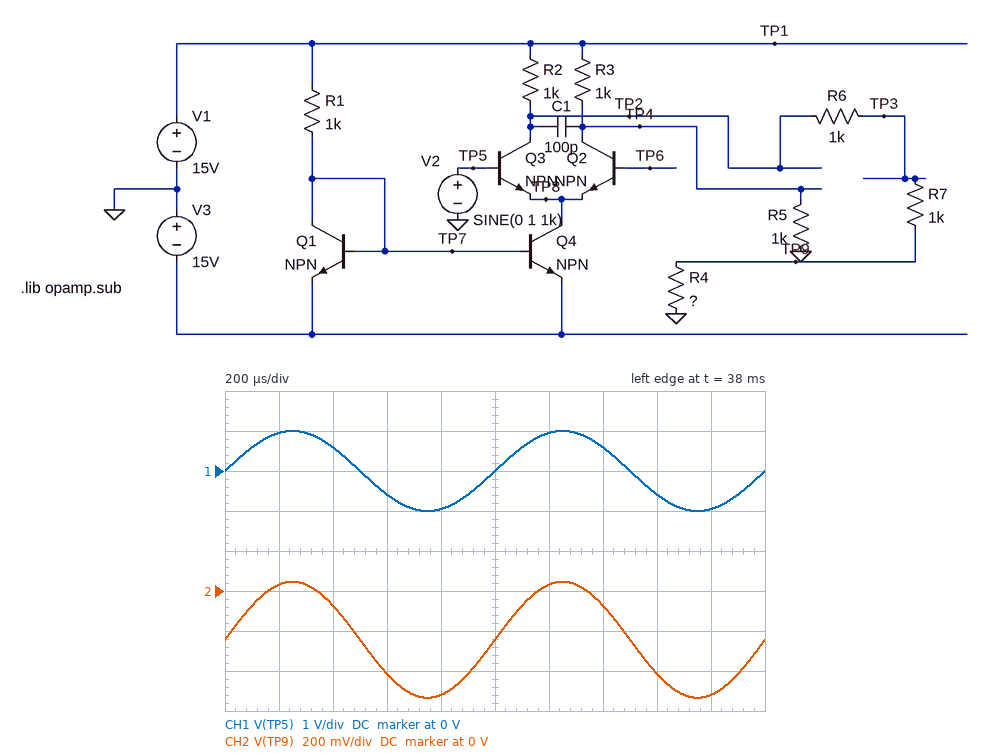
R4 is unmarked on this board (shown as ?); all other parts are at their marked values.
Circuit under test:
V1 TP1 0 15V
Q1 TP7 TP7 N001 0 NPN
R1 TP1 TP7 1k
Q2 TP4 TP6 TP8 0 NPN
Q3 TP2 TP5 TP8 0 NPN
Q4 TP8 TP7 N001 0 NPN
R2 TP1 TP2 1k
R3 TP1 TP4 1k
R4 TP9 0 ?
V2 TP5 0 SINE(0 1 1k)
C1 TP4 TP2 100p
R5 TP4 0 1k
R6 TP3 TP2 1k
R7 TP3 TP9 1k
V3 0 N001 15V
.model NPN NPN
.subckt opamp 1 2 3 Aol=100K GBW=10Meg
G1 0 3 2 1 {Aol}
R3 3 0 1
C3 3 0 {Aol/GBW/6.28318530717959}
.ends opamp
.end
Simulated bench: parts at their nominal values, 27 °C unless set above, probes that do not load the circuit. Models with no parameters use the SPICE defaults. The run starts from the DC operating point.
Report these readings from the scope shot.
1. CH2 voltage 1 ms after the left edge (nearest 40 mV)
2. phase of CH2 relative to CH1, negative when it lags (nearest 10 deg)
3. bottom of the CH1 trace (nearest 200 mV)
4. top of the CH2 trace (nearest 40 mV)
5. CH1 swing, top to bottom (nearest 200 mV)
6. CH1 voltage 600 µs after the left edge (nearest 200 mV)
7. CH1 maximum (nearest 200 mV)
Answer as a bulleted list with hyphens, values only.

- -240 mV
- 0 deg
- -1.0 V
- 40 mV
- 2.0 V
- -600 mV
- 1.0 V
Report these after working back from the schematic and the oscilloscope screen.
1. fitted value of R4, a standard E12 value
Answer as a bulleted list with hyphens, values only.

- 820 Ω
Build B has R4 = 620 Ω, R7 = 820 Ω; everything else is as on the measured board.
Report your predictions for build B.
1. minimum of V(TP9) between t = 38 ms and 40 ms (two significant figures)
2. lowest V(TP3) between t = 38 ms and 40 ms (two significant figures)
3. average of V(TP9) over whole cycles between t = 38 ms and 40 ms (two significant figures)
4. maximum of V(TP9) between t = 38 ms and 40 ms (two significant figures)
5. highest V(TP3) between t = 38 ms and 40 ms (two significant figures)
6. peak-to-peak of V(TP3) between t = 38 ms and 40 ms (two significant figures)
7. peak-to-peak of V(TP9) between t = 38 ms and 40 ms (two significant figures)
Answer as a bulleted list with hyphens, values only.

- -470 mV
- -1.1 V
- -210 mV
- 40 mV
- 94 mV
- 1.2 V
- 510 mV
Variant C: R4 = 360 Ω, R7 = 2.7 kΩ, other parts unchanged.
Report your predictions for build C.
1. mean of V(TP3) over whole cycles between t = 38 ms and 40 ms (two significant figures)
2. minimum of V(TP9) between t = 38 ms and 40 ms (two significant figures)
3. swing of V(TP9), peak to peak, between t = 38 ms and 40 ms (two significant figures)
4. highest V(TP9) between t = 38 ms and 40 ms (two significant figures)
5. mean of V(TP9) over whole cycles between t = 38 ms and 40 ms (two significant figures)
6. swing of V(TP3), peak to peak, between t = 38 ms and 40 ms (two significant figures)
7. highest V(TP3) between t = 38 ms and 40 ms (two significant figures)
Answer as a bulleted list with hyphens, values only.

- -630 mV
- -160 mV
- 180 mV
- 14 mV
- -74 mV
- 1.5 V
- 120 mV
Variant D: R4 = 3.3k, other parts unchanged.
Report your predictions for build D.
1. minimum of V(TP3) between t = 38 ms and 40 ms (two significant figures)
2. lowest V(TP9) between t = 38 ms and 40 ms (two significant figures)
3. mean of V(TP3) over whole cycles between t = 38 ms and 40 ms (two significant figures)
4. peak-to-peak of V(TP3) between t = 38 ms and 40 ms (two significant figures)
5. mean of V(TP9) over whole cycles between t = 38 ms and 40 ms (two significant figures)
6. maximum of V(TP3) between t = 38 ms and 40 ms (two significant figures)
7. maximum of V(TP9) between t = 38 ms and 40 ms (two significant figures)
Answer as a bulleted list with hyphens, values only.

- -1.5 V
- -1.1 V
- -680 mV
- 1.6 V
- -520 mV
- 130 mV
- 99 mV
